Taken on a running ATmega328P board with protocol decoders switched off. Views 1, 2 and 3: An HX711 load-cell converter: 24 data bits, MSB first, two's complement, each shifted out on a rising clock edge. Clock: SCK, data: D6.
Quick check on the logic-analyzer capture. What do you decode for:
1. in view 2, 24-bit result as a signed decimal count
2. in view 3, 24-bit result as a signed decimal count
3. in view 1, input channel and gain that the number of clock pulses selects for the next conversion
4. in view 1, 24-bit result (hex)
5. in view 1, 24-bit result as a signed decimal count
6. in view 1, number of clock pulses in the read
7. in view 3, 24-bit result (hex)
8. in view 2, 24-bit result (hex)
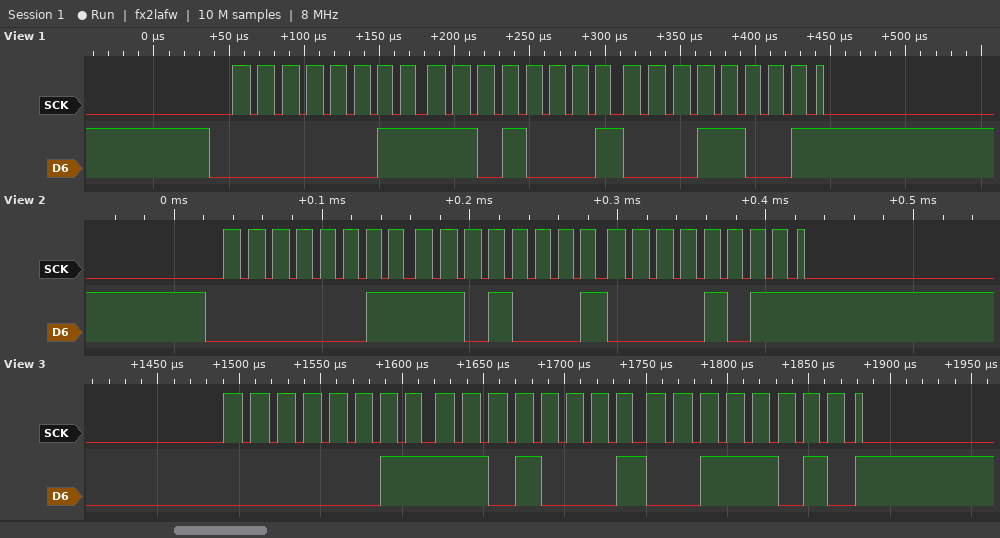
250123
250170
channel A, gain 128
0x03D119
250137
25
0x03D13A
0x03D10B
